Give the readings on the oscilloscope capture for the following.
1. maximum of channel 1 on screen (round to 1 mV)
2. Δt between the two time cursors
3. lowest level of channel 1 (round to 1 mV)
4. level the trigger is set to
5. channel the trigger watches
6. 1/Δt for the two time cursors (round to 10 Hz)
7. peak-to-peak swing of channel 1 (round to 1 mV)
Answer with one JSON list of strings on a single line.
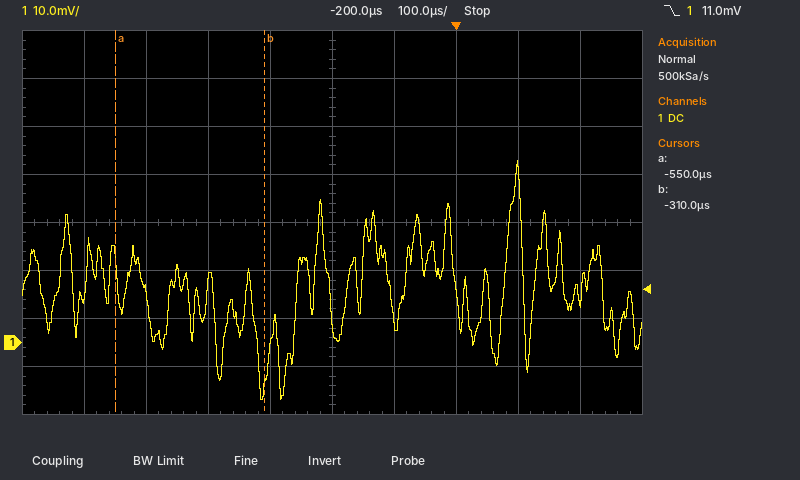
["38 mV", "240 µs", "-12 mV", "11.0 mV", "channel 1", "4.17 kHz", "50 mV"]
